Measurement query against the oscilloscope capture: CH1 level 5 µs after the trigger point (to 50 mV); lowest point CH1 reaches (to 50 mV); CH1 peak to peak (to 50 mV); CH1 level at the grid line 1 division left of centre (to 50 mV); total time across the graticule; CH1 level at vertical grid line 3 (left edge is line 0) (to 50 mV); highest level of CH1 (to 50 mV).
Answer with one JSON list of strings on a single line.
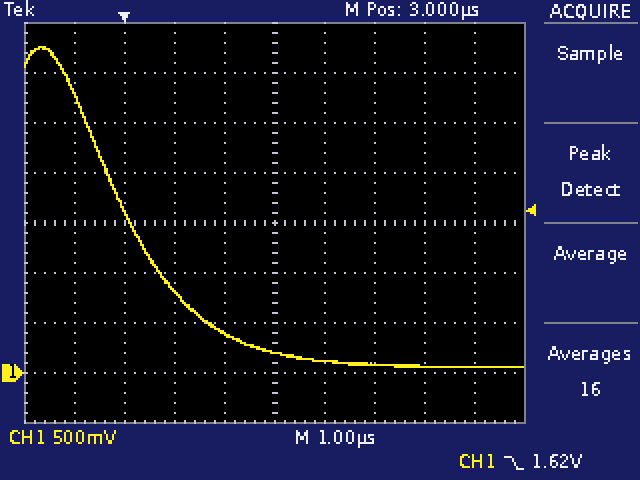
["100 mV", "50 mV", "3.20 V", "400 mV", "10 µs", "800 mV", "3.25 V"]
